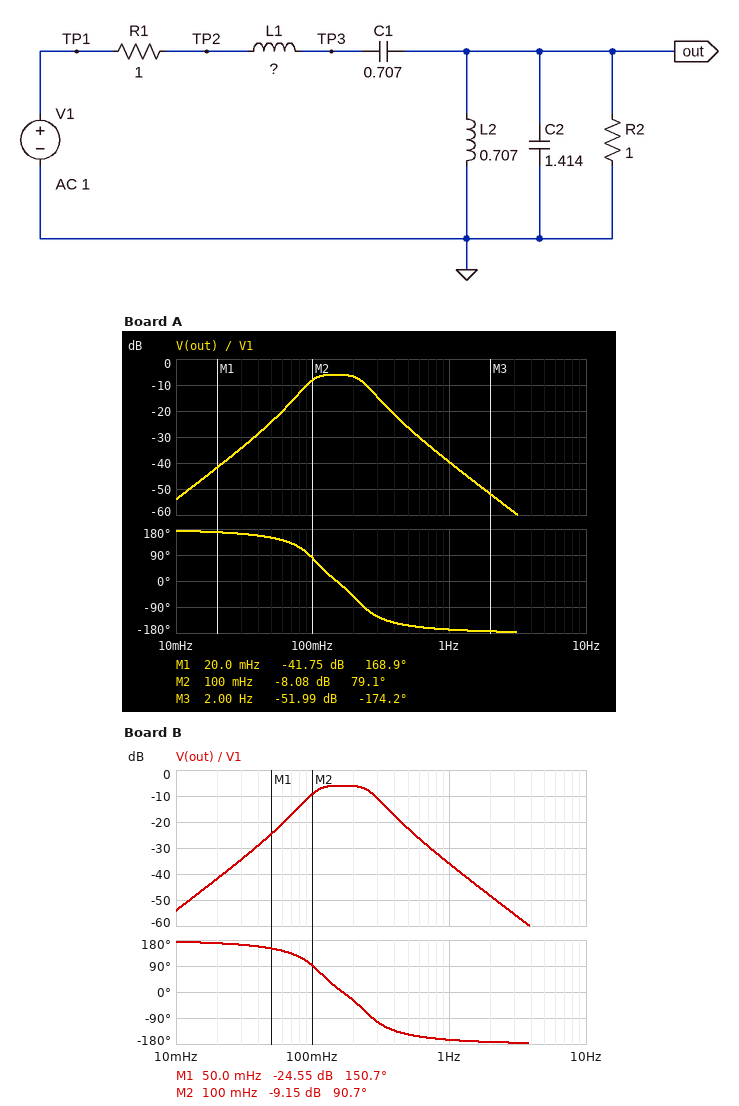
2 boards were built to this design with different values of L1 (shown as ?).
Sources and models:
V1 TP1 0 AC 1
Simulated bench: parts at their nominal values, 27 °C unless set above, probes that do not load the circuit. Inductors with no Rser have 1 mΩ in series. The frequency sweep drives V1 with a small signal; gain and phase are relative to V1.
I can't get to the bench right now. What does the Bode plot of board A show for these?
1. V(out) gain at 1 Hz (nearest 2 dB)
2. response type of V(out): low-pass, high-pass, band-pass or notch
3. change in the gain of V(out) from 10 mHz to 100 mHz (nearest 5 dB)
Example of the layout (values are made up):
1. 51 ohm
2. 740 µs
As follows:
1. -40 dB
2. band-pass
3. 45 dB
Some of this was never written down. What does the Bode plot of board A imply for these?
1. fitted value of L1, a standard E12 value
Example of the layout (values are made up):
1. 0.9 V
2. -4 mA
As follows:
1. 1.8 H
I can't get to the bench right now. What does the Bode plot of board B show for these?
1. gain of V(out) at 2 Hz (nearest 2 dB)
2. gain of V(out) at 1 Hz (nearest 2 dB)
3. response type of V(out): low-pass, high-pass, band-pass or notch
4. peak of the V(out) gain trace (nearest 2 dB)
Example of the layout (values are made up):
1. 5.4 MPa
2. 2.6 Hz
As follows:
1. -48 dB
2. -36 dB
3. band-pass
4. -6 dB
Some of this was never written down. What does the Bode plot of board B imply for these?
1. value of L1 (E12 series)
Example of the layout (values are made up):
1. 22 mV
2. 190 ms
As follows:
1. 1.2 H
